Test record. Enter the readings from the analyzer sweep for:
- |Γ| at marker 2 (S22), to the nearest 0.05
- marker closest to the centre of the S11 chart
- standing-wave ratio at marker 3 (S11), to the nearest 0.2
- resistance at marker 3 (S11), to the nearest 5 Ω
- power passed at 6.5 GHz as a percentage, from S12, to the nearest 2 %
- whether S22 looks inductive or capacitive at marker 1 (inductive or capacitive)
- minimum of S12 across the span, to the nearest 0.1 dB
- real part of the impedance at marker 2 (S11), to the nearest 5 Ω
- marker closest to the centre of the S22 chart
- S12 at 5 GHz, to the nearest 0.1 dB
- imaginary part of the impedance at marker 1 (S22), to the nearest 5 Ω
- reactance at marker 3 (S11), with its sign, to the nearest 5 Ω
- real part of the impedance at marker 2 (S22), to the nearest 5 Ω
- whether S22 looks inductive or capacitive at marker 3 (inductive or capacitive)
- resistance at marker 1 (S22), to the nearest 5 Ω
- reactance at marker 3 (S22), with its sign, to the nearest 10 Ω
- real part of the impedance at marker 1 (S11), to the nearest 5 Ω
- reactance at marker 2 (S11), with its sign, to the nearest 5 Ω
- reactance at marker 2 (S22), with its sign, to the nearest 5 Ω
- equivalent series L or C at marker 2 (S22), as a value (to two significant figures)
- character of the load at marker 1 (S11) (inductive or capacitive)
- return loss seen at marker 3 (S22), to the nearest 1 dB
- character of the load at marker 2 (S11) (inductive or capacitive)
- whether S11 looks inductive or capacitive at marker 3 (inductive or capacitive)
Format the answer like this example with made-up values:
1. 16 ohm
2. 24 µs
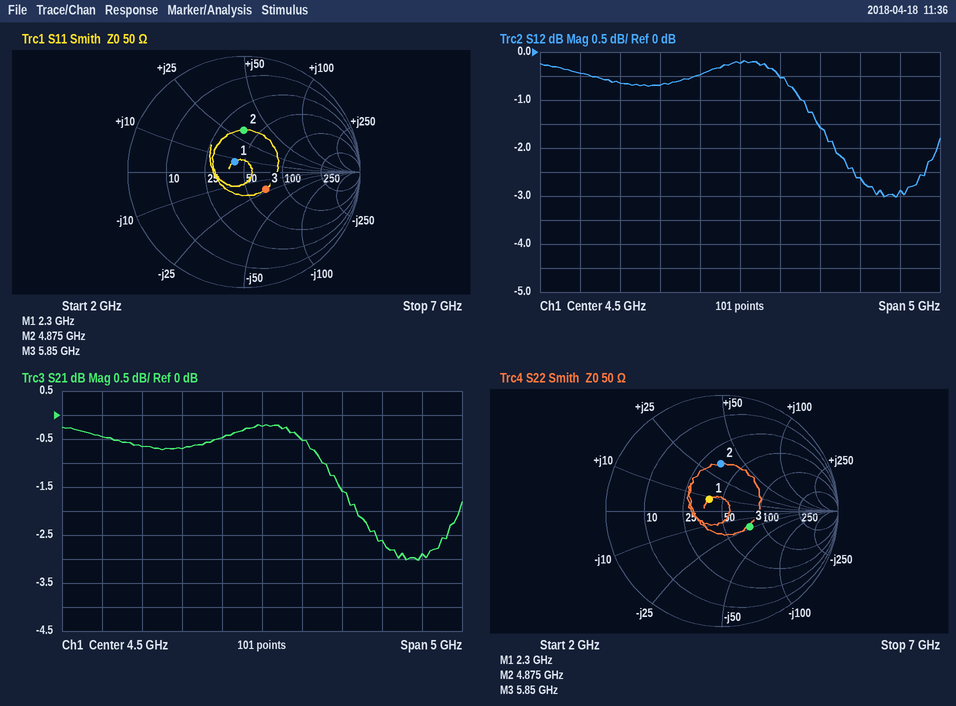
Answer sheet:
1. 0.40
2. marker 1
3. 1.6
4. 70 Ω
5. 52 %
6. inductive
7. -3.0 dB
8. 40 Ω
9. marker 1
10. -0.5 dB
11. +10 Ω
12. -20 Ω
13. 35 Ω
14. capacitive
15. 40 Ω
16. -20 Ω
17. 40 Ω
18. +30 Ω
19. +35 Ω
20. 1.1 nH
21. inductive
22. 11 dB
23. inductive
24. capacitive
